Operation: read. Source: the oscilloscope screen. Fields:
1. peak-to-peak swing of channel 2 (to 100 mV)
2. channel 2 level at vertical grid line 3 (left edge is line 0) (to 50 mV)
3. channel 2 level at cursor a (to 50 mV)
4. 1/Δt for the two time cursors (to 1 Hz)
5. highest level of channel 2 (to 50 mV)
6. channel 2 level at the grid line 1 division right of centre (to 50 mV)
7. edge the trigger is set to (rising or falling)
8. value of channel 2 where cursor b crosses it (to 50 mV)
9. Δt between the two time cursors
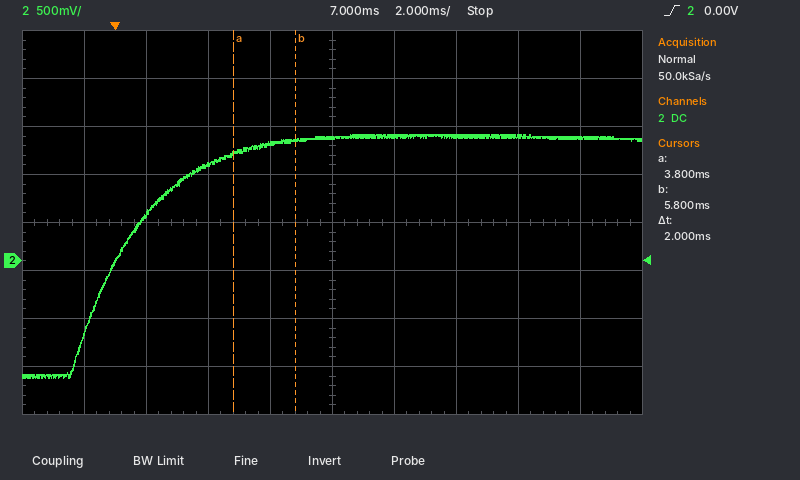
2.50 V
1.00 V
1.10 V
500 Hz
1.30 V
1.30 V
rising
1.25 V
2 ms
